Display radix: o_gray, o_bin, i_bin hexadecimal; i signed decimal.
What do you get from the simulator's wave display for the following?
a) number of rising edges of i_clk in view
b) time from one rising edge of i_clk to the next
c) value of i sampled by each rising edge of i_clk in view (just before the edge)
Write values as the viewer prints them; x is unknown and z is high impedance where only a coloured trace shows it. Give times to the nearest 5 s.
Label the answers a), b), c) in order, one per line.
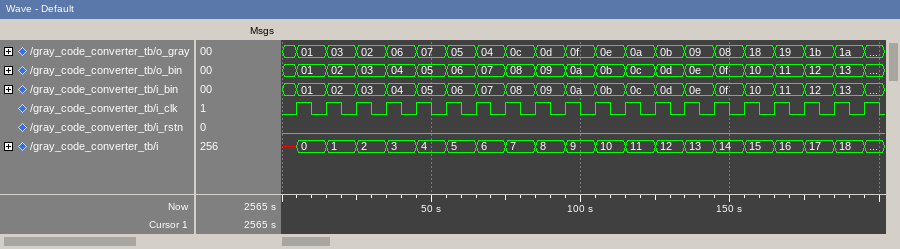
a) 20
b) 10 s
c) x, 0, 1, 2, 3, 4, 5, 6, 7, 8, 9, 10, 11, 12, 13, 14, 15, 16, 17, 18
